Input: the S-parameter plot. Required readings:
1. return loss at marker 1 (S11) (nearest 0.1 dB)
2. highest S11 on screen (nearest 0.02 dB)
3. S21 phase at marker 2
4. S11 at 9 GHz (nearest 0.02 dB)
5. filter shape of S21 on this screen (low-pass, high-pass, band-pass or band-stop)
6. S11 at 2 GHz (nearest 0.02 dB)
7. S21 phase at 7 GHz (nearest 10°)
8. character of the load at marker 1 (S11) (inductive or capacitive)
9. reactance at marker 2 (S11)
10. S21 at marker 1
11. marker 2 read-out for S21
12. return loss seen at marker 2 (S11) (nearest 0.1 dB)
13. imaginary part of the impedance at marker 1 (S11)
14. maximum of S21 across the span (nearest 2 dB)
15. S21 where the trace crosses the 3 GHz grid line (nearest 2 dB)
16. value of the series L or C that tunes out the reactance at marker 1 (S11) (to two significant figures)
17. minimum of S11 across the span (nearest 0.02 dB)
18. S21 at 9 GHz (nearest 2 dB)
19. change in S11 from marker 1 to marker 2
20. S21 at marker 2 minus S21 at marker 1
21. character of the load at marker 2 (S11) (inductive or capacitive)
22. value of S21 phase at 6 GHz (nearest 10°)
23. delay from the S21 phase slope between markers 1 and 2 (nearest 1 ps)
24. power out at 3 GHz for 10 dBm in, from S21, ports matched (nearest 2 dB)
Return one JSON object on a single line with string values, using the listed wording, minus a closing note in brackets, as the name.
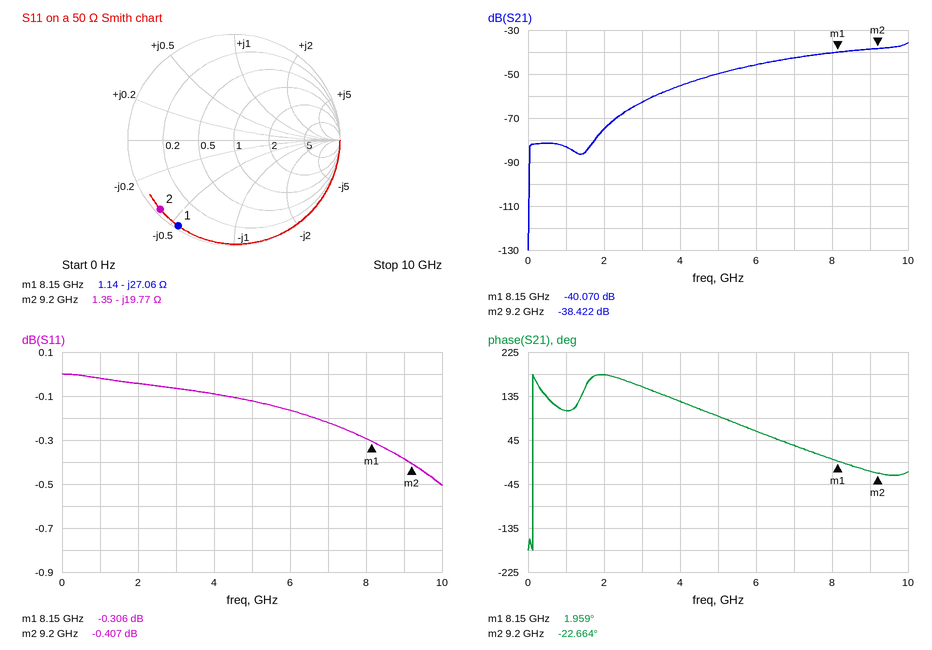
{"return loss at marker 1 (S11)": "0.3 dB", "highest S11 on screen": "0.00 dB", "S21 phase at marker 2": "-22.664°", "S11 at 9 GHz": "-0.38 dB", "filter shape of S21 on this screen": "high-pass", "S11 at 2 GHz": "-0.04 dB", "S21 phase at 7 GHz": "30°", "character of the load at marker 1 (S11)": "capacitive", "reactance at marker 2": "-19.77 Ω", "S21 at marker 1": "-40.070 dB", "marker 2 read-out for S21": "-38.422 dB", "return loss seen at marker 2 (S11)": "0.4 dB", "imaginary part of the impedance at marker 1": "-27.06 Ω", "maximum of S21 across the span": "-36 dB", "S21 where the trace crosses the 3 GHz grid line": "-62 dB", "value of the series L or C that tunes out the reactance at marker 1 (S11)": "530 pH", "minimum of S11 across the span": "-0.50 dB", "S21 at 9 GHz": "-38 dB", "change in S11 from marker 1 to marker 2": "-0.101 dB", "S21 at marker 2 minus S21 at marker 1": "1.648 dB", "character of the load at marker 2 (S11)": "capacitive", "value of S21 phase at 6 GHz": "60°", "delay from the S21 phase slope between markers 1 and 2": "65 ps", "power out at 3 GHz for 10 dBm in, from S21, ports matched": "-52 dBm"}
